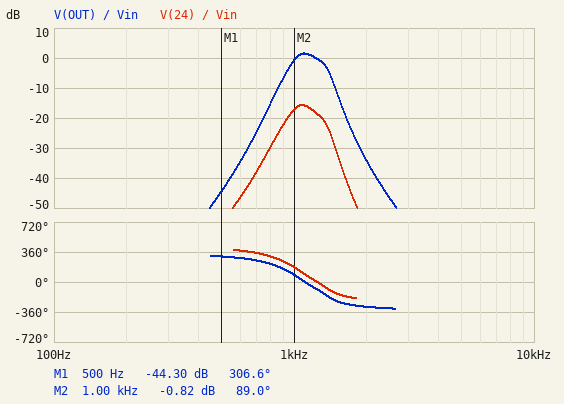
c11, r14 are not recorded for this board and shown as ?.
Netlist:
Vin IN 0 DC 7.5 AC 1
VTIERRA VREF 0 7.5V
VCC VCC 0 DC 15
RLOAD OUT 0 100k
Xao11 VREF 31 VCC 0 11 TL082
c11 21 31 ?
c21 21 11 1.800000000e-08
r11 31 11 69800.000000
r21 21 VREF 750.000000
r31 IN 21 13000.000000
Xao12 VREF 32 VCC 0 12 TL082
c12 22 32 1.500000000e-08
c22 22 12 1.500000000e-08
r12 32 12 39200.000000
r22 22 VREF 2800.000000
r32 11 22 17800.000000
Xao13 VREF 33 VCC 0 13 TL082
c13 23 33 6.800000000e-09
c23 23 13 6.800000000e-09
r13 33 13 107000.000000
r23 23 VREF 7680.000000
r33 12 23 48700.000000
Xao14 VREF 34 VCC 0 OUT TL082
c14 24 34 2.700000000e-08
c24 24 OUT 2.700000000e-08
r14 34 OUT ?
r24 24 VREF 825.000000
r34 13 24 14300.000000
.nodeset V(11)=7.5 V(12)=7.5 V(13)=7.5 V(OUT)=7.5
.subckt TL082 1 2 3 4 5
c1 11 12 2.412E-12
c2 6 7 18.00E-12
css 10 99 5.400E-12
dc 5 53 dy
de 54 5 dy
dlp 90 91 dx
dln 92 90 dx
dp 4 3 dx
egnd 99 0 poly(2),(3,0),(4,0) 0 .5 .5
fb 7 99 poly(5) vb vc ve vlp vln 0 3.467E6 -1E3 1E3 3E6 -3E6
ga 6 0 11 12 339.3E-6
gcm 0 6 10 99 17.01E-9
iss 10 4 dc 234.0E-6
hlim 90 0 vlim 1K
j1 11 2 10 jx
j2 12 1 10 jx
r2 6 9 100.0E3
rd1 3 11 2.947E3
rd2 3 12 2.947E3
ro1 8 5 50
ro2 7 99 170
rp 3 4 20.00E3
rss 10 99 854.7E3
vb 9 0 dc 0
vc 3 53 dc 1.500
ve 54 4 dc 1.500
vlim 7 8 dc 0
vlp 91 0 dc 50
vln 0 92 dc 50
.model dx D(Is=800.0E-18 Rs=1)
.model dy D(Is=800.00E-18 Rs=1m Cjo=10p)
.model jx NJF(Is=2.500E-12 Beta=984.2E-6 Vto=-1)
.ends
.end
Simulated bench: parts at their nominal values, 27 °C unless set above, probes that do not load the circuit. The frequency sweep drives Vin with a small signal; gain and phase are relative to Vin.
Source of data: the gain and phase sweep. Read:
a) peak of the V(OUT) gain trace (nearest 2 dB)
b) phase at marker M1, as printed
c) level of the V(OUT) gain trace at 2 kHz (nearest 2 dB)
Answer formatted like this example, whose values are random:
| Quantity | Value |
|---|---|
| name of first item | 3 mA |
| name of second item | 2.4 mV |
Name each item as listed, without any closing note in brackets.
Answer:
| Quantity | Value |
|---|---|
| peak of the V(OUT) gain trace | 2 dB |
| phase at marker M1, as printed | 306.6 deg |
| level of the V(OUT) gain trace at 2 kHz | -34 dB |
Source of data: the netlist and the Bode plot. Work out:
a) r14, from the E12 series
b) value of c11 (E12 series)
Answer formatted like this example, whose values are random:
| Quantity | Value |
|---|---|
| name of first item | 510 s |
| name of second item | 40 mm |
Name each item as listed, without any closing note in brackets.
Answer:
| Quantity | Value |
|---|---|
| r14, from the E12 series | 39 kΩ |
| value of c11 | 15 nF |
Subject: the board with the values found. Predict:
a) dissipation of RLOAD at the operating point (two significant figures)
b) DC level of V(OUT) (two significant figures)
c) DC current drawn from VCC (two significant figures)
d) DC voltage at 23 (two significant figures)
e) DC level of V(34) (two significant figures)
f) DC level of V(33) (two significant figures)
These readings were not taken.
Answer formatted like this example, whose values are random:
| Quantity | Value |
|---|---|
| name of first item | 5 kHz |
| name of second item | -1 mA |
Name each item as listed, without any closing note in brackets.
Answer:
| Quantity | Value |
|---|---|
| dissipation of RLOAD at the operating point | 560 µW |
| DC level of V(OUT) | 7.5 V |
| DC current drawn from VCC | 3.9 mA |
| DC voltage at 23 | 7.5 V |
| DC level of V(34) | 7.5 V |
| DC level of V(33) | 7.5 V |
